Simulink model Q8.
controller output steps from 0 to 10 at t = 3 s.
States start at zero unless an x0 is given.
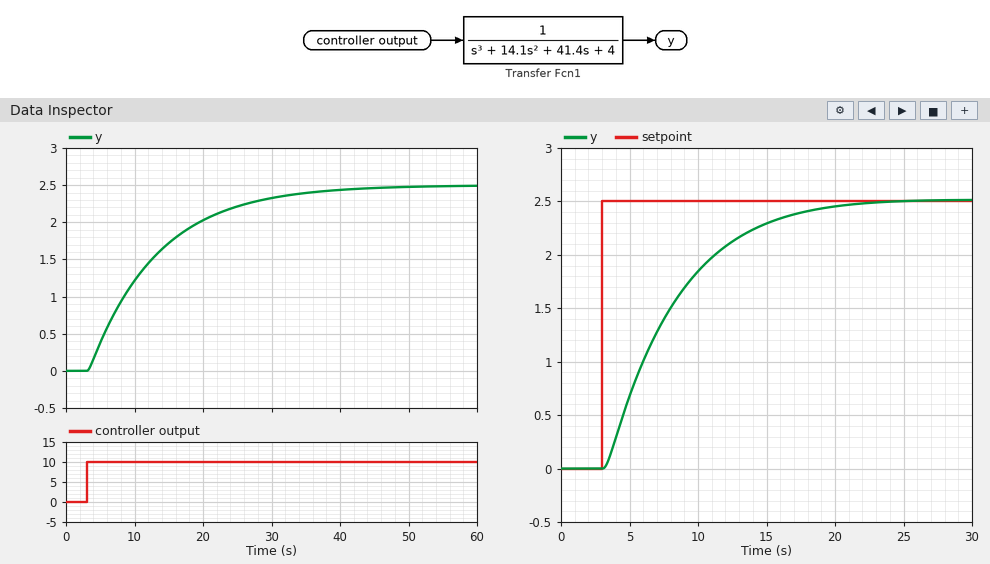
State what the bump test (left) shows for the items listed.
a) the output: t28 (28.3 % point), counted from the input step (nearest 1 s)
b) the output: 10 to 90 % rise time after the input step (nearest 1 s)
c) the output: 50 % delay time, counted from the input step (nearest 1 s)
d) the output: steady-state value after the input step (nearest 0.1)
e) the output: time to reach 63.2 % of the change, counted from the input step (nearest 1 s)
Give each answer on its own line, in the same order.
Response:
4 s
22 s
7 s
2.5
10 s
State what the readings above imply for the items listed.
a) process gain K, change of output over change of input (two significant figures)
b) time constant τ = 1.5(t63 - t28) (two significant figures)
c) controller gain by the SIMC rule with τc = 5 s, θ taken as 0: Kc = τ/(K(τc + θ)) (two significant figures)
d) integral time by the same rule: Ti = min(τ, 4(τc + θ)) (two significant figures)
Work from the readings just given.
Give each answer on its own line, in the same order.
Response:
0.25
9.0 s
7.2
9.0 s
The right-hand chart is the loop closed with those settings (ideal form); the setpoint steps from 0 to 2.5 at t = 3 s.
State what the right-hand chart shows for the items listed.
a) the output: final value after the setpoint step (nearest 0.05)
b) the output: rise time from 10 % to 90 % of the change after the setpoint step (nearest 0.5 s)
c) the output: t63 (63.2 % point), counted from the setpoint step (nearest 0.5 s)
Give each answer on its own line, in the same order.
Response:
2.50
10.5 s
5.5 s
